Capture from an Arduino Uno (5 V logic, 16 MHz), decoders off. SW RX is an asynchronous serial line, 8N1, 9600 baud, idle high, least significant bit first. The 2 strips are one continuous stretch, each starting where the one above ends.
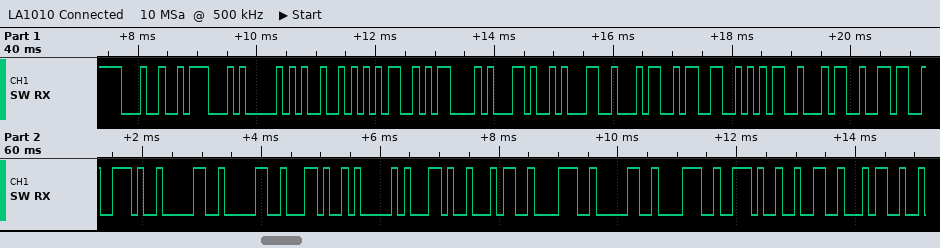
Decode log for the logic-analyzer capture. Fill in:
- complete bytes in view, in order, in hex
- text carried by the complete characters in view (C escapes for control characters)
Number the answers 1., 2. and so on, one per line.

1. 24 47 50 52 4D 43 2C 31 34 33 35 34 36 2E 30 30 2C 41 2C 34 38 30 38 2E 32 34
2. "$GPRMC,143546.00,A,4808.24"
